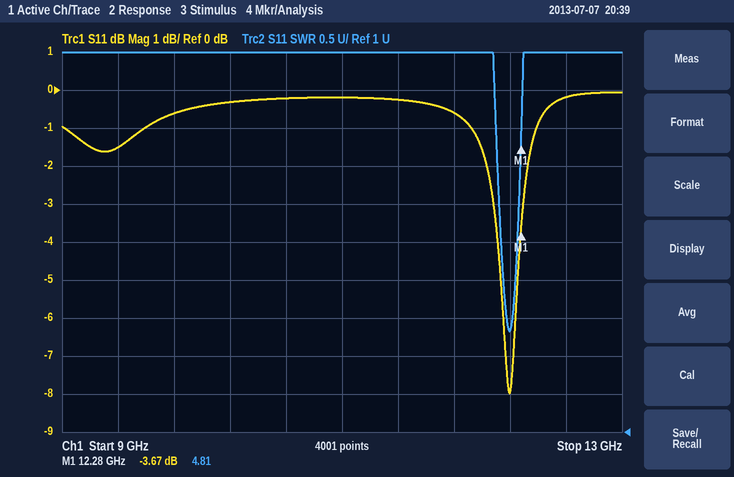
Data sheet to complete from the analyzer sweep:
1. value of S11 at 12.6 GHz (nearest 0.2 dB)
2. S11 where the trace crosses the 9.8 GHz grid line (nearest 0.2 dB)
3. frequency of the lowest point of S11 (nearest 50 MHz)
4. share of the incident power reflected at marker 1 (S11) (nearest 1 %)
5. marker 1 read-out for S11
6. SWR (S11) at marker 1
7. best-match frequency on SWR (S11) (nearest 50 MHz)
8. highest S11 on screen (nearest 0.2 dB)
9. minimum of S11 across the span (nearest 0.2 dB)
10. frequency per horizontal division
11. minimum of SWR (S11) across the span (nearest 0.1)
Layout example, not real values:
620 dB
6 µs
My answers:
-0.2 dB
-0.6 dB
12.20 GHz
43 %
-3.67 dB
4.81
12.20 GHz
0.0 dB
-8.0 dB
400 MHz
2.3
